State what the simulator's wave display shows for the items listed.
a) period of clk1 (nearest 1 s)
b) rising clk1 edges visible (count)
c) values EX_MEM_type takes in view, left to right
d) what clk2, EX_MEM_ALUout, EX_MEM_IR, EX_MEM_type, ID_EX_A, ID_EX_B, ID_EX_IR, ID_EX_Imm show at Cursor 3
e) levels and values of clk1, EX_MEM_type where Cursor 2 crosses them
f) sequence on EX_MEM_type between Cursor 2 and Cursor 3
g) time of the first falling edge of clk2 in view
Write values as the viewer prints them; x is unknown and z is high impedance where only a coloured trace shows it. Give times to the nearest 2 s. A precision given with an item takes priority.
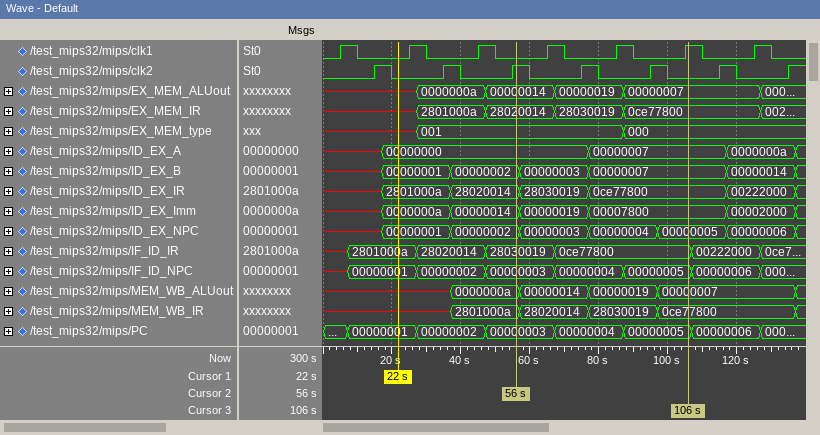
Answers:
20 s
7
x, 001, 000
clk2=0, EX_MEM_ALUout=00000007, EX_MEM_IR=0ce77800, EX_MEM_type=000, ID_EX_A=00000007, ID_EX_B=00000007, ID_EX_IR=0ce77800, ID_EX_Imm=00007800
clk1=0, EX_MEM_type=001
001, 000
20 s
